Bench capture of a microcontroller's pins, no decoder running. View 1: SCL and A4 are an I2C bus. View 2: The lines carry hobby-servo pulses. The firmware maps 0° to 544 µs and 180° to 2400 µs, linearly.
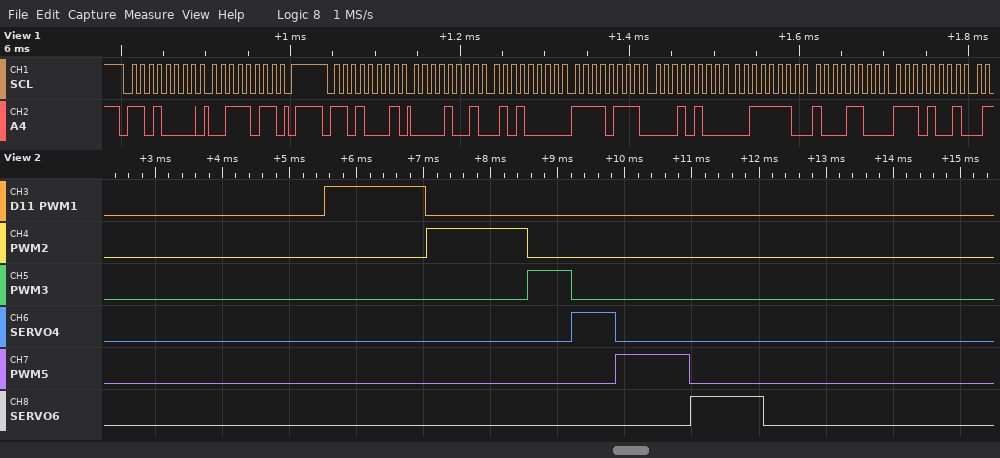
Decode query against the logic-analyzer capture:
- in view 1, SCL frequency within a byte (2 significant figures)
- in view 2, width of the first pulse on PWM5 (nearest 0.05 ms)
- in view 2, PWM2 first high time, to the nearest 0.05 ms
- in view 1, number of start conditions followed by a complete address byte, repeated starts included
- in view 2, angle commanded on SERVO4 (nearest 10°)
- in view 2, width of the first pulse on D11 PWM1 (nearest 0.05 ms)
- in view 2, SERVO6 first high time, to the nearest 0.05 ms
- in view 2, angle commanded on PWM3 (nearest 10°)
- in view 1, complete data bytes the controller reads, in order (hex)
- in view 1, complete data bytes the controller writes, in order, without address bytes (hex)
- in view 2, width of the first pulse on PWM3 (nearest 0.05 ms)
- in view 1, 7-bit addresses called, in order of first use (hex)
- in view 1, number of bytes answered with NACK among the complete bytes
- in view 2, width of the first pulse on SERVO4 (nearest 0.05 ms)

100 kHz
1.10 ms
1.50 ms
2
10°
1.50 ms
1.10 ms
10°
09 50 F7 14 3E 8C E9
3B
0.65 ms
0x68
0
0.65 ms
